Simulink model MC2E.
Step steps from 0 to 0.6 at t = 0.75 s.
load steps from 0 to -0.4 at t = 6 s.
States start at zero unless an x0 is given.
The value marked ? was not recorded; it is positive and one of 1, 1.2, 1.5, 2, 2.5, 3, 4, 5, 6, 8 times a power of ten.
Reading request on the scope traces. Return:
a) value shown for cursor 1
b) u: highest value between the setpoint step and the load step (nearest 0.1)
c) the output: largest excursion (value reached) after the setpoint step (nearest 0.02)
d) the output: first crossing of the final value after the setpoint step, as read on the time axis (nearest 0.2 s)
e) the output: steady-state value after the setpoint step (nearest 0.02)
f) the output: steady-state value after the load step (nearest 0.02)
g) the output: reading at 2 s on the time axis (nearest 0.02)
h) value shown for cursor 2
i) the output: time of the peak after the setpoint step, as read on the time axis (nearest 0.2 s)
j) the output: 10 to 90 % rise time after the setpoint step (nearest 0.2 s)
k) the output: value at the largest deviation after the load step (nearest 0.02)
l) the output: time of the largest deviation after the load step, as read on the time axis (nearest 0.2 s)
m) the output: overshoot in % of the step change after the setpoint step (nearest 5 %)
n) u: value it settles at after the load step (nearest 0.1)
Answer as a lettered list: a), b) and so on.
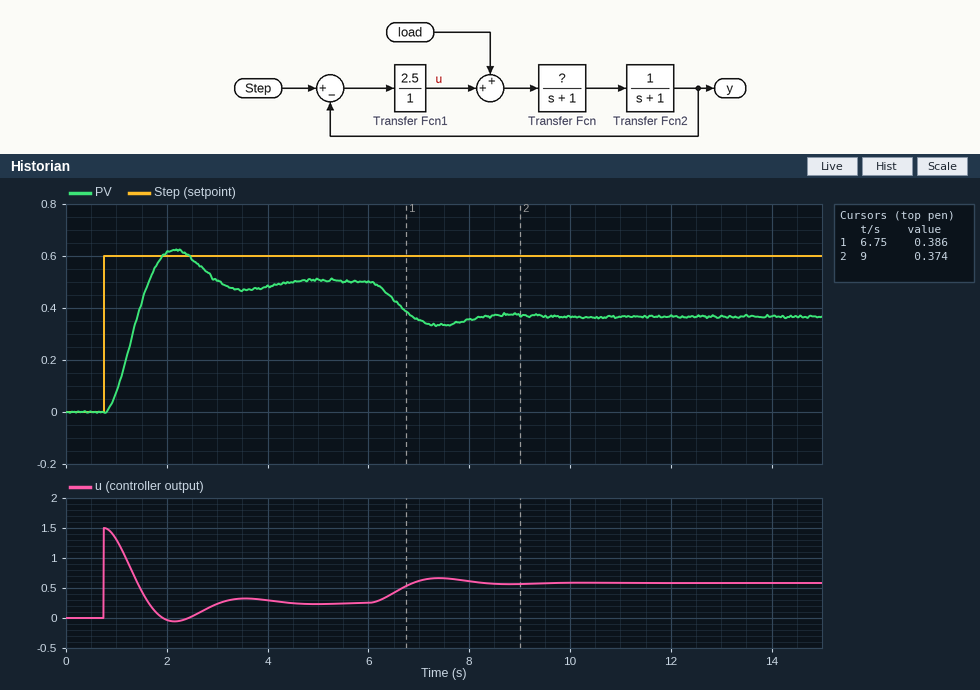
a) 0.386
b) 1.5
c) 0.62
d) 1.6 s
e) 0.50
f) 0.36
g) 0.62
h) 0.374
i) 2.2 s
j) 0.6 s
k) 0.34
l) 7.4 s
m) 25 %
n) 0.6
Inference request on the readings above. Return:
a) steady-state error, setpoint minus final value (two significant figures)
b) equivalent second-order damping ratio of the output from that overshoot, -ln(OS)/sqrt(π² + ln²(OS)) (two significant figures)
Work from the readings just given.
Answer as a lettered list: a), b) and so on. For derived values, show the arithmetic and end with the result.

a) 0.6 - 0.5 = 0.10
b) ln(0.25) = -1.386; 1.386 / sqrt(9.870 + 1.922) = 0.40
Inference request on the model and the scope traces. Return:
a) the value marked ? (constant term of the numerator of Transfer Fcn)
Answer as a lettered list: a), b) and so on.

a) 2
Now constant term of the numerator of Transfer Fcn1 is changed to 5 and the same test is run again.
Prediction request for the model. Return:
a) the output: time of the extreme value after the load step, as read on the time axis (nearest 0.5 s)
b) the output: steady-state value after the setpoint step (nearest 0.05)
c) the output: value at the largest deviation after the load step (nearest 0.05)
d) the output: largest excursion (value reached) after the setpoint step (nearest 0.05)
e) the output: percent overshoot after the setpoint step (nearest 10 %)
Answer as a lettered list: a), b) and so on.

a) 7.0 s
b) 0.55
c) 0.45
d) 0.75
e) 40 %
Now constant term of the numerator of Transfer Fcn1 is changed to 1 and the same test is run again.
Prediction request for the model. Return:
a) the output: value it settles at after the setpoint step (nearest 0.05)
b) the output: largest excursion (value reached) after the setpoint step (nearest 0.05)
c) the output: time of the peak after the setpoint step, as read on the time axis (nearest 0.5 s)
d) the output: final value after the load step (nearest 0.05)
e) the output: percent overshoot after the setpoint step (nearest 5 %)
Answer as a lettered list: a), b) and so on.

a) 0.40
b) 0.45
c) 3.0 s
d) 0.15
e) 10 %
